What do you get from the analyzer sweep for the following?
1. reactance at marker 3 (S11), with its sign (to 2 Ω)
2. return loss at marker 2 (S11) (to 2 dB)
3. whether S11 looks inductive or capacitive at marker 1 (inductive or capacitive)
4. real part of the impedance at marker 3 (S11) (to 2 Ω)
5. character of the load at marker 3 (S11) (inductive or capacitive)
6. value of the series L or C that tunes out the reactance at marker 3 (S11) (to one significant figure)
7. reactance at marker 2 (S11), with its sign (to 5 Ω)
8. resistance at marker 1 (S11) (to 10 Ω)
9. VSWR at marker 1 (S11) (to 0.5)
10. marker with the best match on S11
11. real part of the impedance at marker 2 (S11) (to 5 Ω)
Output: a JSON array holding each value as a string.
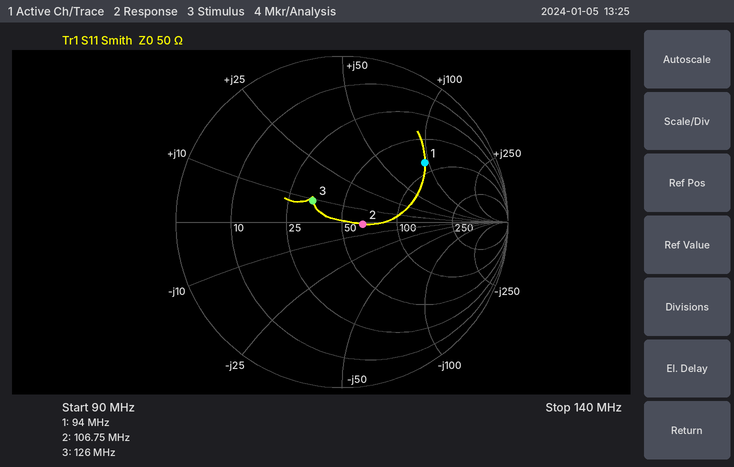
["+10 Ω", "18 dB", "inductive", "34 Ω", "inductive", "100 pF", "0 Ω", "80 Ω", "4.0", "marker 2", "65 Ω"]
